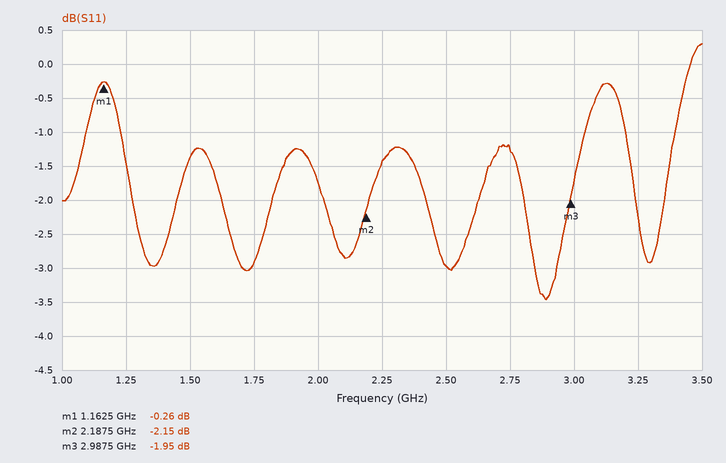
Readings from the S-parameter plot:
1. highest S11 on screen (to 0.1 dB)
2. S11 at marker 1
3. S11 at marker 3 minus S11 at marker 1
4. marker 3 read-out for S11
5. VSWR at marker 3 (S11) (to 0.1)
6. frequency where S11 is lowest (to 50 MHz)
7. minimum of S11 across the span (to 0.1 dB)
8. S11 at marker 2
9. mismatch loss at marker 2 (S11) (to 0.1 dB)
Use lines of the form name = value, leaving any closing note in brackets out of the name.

highest S11 on screen = 0.3 dB
S11 at marker 1 = -0.26 dB
S11 at marker 3 minus S11 at marker 1 = -1.69 dB
marker 3 read-out for S11 = -1.95 dB
VSWR at marker 3 (S11) = 8.9
frequency where S11 is lowest = 2.90 GHz
minimum of S11 across the span = -3.5 dB
S11 at marker 2 = -2.15 dB
mismatch loss at marker 2 (S11) = 4.1 dB
